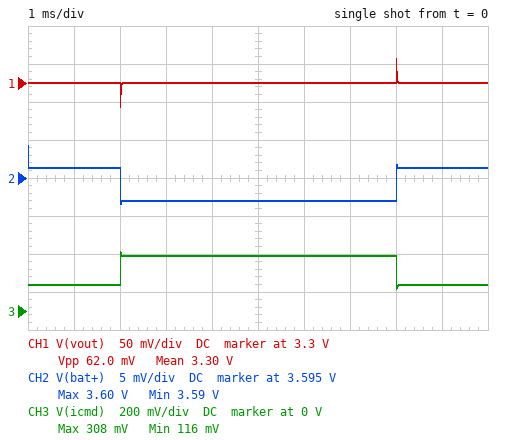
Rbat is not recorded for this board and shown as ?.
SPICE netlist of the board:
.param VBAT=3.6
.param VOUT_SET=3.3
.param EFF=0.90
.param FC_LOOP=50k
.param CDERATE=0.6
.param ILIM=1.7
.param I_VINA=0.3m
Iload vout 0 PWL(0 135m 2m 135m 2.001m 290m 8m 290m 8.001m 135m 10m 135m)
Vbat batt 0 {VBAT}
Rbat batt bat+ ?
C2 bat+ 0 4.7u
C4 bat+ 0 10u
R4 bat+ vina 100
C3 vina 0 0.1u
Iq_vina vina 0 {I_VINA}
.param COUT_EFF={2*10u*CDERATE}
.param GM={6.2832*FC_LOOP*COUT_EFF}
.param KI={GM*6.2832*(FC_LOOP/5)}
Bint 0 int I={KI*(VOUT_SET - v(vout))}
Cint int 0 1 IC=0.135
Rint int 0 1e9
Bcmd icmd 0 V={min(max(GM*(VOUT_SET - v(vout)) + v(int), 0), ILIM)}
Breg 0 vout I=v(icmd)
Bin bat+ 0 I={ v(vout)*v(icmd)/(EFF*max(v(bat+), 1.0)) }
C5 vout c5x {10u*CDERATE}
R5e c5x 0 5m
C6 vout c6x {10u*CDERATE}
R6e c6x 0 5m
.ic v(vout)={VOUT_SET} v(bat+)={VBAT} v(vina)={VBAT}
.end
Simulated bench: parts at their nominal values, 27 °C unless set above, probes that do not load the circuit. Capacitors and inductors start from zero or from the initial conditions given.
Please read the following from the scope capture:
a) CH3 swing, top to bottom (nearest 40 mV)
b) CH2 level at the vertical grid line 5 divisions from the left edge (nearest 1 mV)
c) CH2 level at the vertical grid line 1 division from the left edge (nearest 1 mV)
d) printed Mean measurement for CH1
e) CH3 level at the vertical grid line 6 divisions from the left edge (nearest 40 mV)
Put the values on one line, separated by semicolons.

200 mV; 3.592 V; 3.596 V; 3.30 V; 280 mV
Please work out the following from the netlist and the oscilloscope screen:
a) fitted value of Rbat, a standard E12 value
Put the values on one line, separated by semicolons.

0.027 Ω
